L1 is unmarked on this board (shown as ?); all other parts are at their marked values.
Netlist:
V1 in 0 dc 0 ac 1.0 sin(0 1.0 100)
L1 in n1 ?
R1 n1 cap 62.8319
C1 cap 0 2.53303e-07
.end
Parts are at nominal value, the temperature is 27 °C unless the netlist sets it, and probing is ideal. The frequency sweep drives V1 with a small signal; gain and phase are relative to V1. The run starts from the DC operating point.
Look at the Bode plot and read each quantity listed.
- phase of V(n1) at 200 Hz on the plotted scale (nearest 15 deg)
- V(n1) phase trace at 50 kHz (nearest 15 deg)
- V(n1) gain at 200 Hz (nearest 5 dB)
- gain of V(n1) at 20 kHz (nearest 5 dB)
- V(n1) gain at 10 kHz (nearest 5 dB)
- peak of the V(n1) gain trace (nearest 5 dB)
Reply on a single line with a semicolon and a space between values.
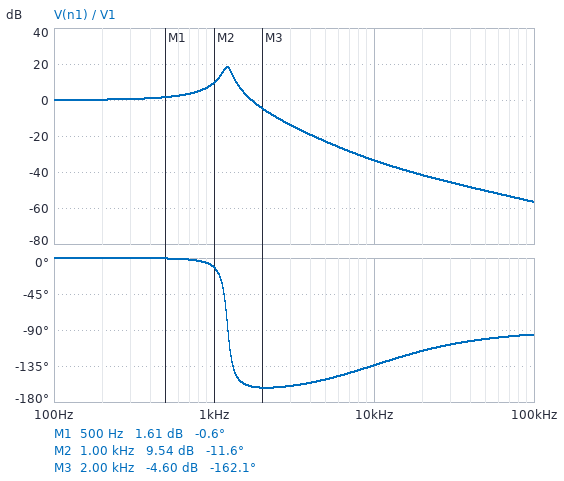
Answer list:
0 deg; -105 deg; 0 dB; -40 dB; -35 dB; 20 dB
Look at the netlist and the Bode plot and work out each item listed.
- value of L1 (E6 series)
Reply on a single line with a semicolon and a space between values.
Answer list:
68 mH
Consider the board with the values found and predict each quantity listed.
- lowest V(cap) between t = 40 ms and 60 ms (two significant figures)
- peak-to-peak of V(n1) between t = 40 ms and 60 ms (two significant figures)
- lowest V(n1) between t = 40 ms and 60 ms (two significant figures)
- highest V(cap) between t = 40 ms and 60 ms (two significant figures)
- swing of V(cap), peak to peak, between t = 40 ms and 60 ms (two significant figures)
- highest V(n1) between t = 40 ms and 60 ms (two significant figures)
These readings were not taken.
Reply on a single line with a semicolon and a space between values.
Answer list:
-1.0 V; 2.0 V; -1.0 V; 1.0 V; 2.0 V; 1.0 V
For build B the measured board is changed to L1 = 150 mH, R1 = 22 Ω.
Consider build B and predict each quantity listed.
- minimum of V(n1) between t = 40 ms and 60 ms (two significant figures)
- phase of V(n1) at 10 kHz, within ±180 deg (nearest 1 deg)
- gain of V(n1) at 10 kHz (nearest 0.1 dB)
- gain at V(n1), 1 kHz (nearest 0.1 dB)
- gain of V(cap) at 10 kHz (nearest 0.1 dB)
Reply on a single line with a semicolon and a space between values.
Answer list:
-1.0 V; -161 deg; -43.0 dB; 6.0 dB; -43.5 dB
